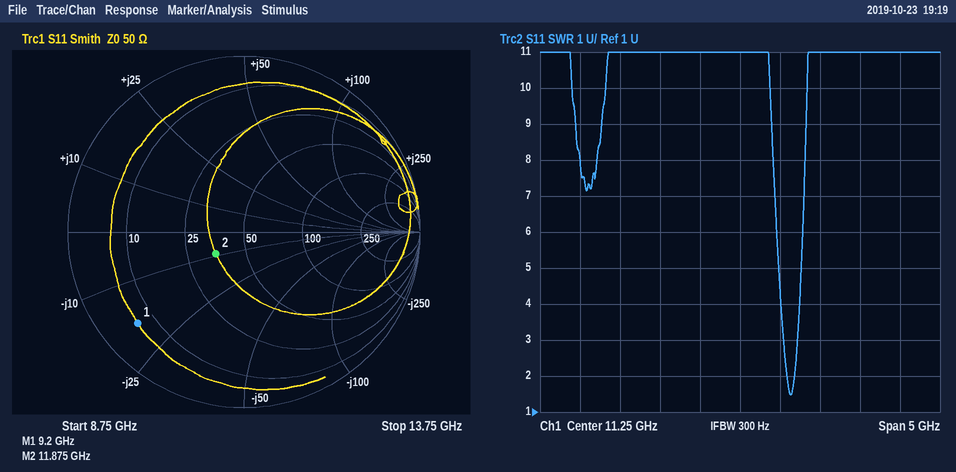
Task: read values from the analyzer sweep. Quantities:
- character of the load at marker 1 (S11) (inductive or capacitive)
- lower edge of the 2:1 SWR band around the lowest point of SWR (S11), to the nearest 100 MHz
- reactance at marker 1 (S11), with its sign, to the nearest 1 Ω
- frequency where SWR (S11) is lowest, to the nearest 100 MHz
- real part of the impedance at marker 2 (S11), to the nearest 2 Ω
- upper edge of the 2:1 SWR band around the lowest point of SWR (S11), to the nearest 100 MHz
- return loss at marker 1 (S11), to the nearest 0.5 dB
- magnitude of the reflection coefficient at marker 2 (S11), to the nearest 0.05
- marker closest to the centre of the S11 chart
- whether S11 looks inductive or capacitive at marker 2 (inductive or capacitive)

capacitive
11.8 GHz
-18 Ω
11.9 GHz
36 Ω
11.9 GHz
2.0 dB
0.20
marker 2
capacitive
